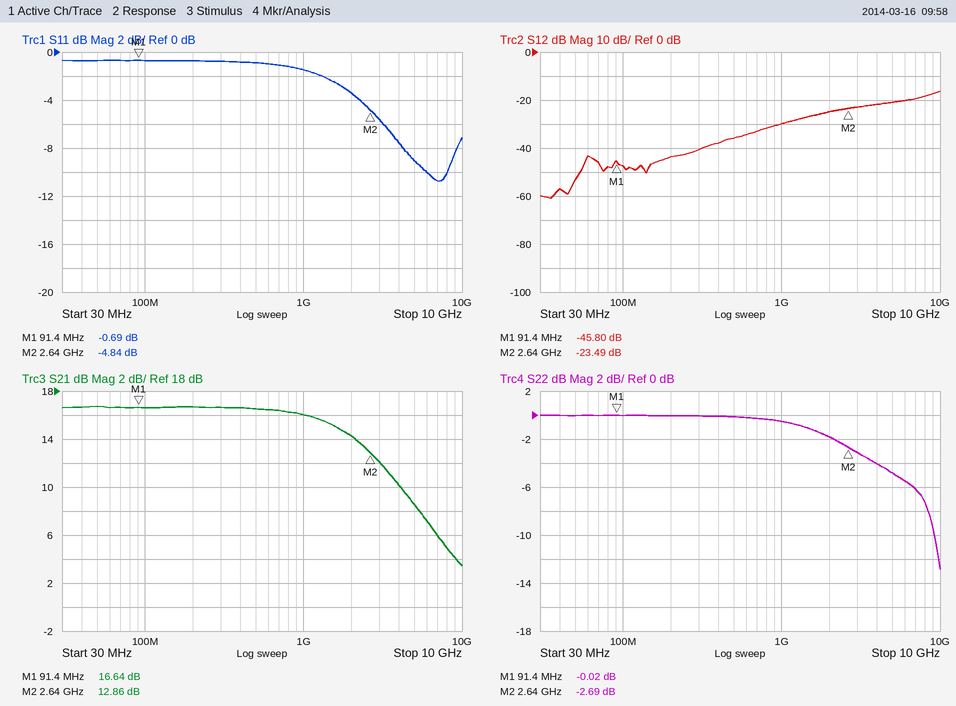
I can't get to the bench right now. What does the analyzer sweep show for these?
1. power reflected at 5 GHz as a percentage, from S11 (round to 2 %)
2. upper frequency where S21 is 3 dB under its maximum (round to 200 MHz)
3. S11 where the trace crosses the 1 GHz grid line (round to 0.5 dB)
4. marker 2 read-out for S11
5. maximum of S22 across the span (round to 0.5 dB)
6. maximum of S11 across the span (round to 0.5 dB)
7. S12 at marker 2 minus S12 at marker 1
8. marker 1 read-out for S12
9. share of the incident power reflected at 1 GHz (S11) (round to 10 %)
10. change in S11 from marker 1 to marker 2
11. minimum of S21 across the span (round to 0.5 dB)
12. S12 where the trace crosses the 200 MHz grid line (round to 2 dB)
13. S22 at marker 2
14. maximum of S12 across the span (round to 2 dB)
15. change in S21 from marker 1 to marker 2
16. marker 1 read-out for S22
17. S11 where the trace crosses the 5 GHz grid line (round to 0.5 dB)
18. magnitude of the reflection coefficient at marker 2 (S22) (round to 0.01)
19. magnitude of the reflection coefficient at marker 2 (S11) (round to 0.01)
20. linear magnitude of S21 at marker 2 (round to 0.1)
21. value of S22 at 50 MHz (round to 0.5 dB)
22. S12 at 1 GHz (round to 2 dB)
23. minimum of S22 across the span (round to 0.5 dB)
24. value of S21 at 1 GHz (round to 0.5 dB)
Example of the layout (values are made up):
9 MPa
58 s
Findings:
12 %
2.2 GHz
-1.5 dB
-4.84 dB
0.0 dB
-0.5 dB
22.31 dB
-45.80 dB
70 %
-4.15 dB
3.5 dB
-44 dB
-2.69 dB
-16 dB
-3.78 dB
-0.02 dB
-9.0 dB
0.73
0.57
4.4
0.0 dB
-30 dB
-13.0 dB
16.0 dB
